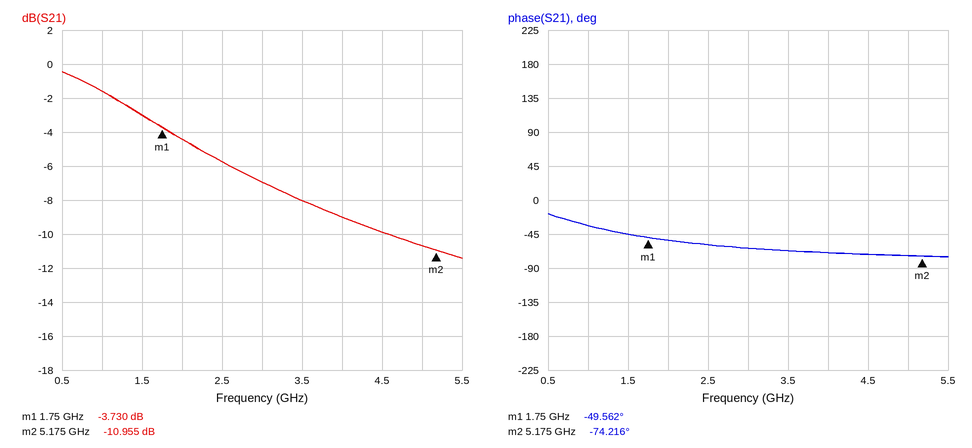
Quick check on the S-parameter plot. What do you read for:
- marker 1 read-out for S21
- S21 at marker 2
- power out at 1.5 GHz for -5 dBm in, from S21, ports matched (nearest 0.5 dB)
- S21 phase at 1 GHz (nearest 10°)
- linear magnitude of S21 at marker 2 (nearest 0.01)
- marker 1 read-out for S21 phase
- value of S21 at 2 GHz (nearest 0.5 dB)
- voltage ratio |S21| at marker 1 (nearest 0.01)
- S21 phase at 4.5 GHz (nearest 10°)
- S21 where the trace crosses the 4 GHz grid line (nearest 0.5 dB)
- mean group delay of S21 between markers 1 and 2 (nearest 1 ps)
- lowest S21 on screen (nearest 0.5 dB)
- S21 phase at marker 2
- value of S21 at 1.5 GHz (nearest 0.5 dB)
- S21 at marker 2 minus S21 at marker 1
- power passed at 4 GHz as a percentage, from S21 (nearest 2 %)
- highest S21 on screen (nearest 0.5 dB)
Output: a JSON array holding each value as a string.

["-3.730 dB", "-10.955 dB", "-8.0 dBm", "-30°", "0.28", "-49.562°", "-4.5 dB", "0.65", "-70°", "-9.0 dB", "20 ps", "-11.5 dB", "-74.216°", "-3.0 dB", "-7.225 dB", "12 %", "-0.5 dB"]
